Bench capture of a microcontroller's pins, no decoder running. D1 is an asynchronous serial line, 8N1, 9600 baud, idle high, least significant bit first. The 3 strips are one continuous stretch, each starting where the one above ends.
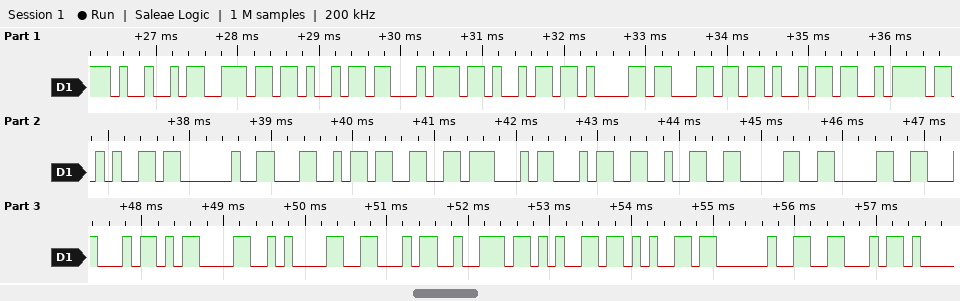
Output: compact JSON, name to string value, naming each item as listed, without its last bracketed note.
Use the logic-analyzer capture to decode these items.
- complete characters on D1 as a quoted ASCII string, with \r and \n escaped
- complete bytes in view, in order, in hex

{"complete characters on D1 as a quoted ASCII string, with \\r and \\n escaped": "\"Initialize L3G4200D\\r\\nFree F\"", "complete bytes in view, in order, in hex": "49 6E 69 74 69 61 6C 69 7A 65 20 4C 33 47 34 32 30 30 44 0D 0A 46 72 65 65 20 46"}
